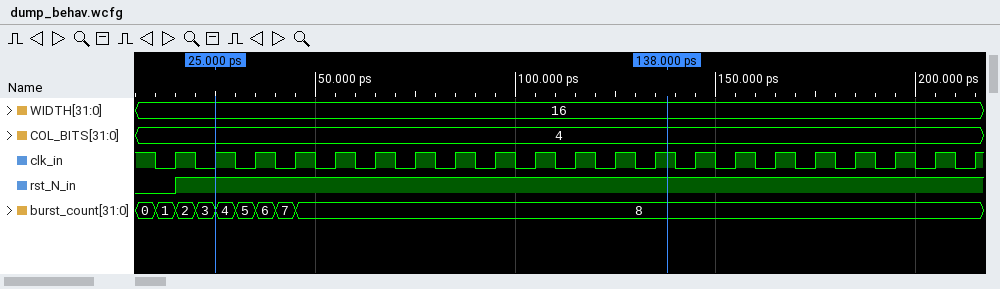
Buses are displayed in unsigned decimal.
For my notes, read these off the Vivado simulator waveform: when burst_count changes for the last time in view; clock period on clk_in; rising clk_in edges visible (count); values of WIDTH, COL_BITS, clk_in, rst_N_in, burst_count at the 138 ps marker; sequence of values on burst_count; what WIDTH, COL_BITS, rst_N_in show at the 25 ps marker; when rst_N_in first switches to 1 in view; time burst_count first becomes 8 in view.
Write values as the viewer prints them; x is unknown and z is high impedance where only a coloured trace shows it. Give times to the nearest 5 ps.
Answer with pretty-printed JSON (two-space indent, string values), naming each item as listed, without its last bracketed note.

{
  "when burst_count changes for the last time in view": "45 ps",
  "clock period on clk_in": "10 ps",
  "rising clk_in edges visible": "21",
  "values of WIDTH, COL_BITS, clk_in, rst_N_in, burst_count at the 138 ps marker": "WIDTH=16, COL_BITS=4, clk_in=1, rst_N_in=1, burst_count=8",
  "sequence of values on burst_count": "0, 1, 2, 3, 4, 5, 6, 7, 8",
  "what WIDTH, COL_BITS, rst_N_in show at the 25 ps marker": "WIDTH=16, COL_BITS=4, rst_N_in=1",
  "when rst_N_in first switches to 1 in view": "15 ps",
  "time burst_count first becomes 8 in view": "45 ps"
}
